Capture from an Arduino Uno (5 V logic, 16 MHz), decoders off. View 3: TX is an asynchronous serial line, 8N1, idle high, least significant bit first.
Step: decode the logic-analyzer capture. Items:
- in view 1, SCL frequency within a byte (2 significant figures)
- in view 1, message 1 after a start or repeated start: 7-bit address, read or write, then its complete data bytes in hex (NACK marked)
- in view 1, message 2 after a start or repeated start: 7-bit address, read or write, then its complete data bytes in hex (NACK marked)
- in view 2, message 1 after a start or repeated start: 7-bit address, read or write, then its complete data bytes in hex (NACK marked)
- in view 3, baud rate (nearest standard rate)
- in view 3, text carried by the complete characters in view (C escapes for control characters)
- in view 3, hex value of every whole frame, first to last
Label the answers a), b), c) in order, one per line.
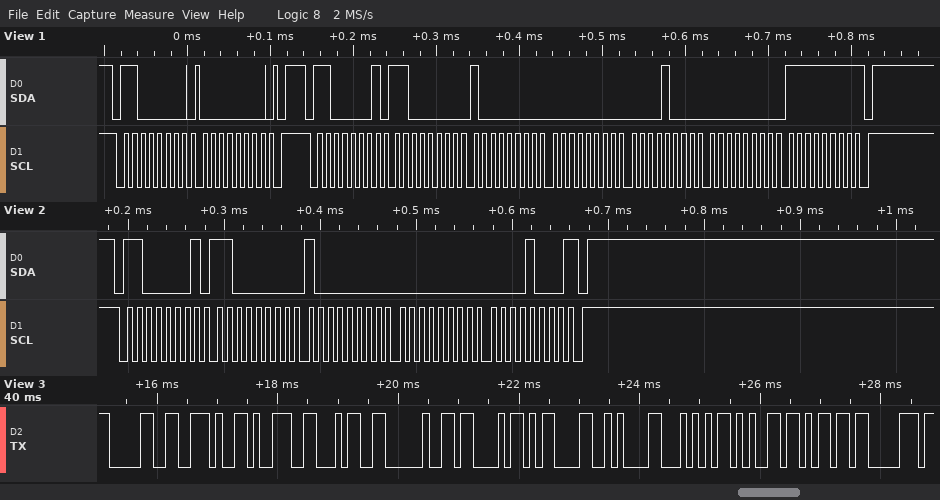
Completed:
a) 100 kHz
b) 0x60 write: 00
c) 0x60 read: C0 80 00 08 00 FF NACK
d) 0x60 read: C0 80 00 08 NACK
e) 9600 baud
f) "0.94 C\r\nTemp"
g) 30 2E 39 34 20 43 0D 0A 54 65 6D 70
